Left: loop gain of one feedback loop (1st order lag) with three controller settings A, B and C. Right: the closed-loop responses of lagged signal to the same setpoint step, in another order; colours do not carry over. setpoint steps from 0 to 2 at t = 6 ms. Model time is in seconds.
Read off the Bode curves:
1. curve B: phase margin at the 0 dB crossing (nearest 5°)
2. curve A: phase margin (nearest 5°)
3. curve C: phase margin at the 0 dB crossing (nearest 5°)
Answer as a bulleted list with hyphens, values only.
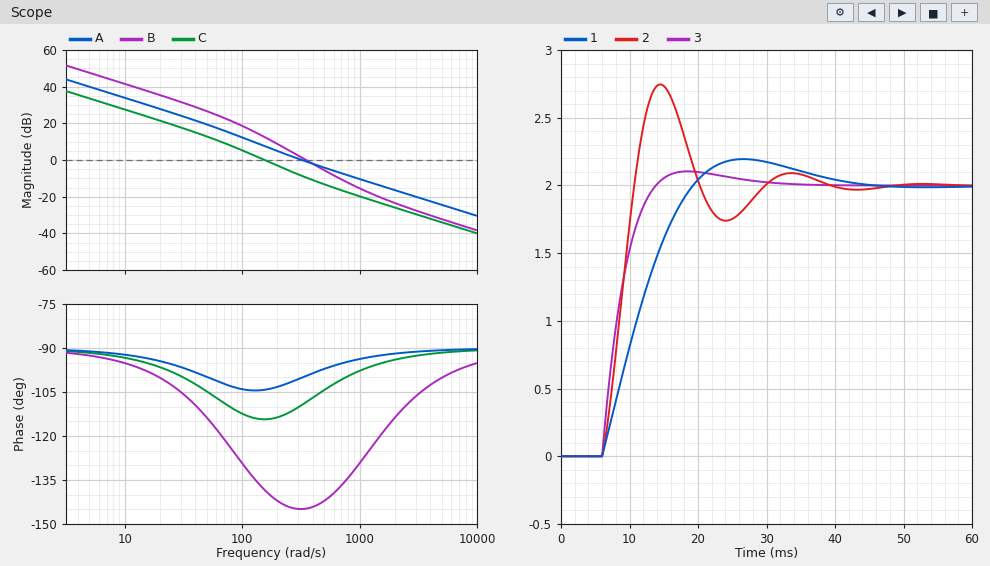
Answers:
- 35°
- 80°
- 65°
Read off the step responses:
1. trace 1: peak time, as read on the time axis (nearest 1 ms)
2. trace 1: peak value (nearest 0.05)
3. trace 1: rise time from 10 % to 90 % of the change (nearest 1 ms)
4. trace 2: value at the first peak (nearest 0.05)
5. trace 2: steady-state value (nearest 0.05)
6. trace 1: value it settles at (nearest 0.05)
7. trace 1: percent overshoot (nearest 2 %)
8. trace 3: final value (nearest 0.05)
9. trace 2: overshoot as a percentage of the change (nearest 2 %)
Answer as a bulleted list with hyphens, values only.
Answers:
- 27 ms
- 2.20
- 10 ms
- 2.75
- 2.00
- 2.00
- 10 %
- 2.00
- 38 %
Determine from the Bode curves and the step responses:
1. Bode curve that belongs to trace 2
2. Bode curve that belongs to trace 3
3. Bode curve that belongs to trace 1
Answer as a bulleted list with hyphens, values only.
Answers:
- B
- A
- C
